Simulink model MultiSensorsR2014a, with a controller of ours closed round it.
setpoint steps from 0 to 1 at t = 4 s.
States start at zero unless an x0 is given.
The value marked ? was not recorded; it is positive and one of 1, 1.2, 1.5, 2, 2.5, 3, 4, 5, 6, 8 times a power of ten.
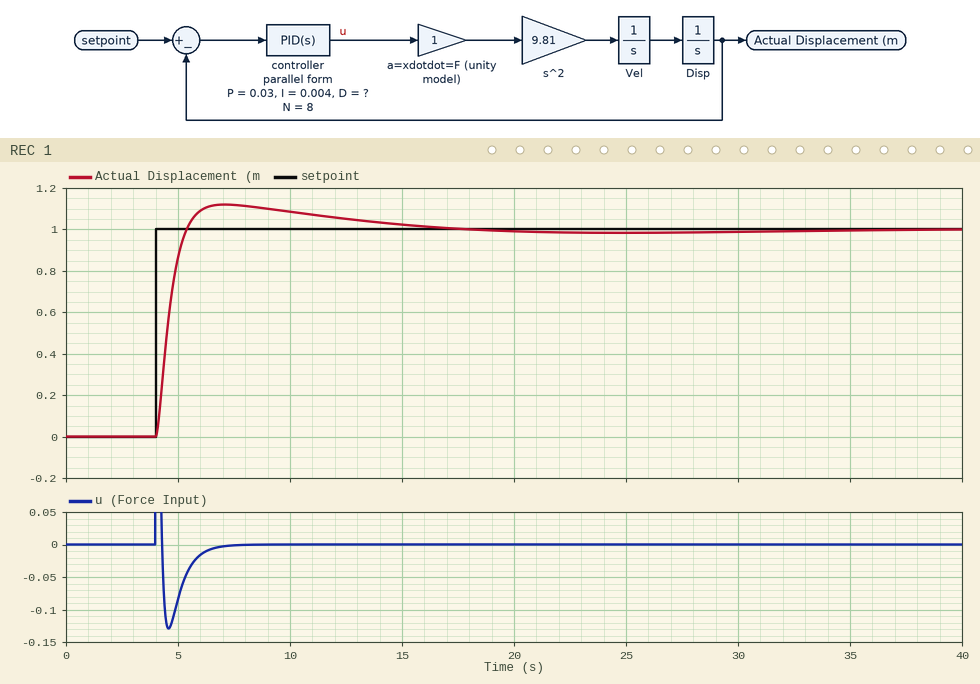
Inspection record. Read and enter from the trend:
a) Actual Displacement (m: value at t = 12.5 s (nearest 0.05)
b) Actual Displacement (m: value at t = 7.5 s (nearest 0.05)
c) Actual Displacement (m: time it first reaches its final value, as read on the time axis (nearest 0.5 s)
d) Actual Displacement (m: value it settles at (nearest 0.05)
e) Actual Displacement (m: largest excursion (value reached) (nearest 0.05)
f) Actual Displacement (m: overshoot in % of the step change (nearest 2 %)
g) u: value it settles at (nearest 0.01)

1.05
1.10
5.5 s
1.00
1.10
12 %
0.00
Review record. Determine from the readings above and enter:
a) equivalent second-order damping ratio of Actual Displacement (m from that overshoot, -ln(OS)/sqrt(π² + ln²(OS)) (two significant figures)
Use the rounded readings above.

0.56
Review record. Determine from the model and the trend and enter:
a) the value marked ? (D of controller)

0.15
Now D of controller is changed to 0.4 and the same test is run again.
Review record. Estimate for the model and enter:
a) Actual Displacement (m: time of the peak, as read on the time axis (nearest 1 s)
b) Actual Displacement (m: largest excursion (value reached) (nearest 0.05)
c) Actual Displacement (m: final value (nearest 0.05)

5 s
1.05
1.00
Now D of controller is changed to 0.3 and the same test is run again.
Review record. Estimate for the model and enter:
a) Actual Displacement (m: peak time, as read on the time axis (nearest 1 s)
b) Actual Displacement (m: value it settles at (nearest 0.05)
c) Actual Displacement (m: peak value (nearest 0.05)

5 s
1.00
1.05
